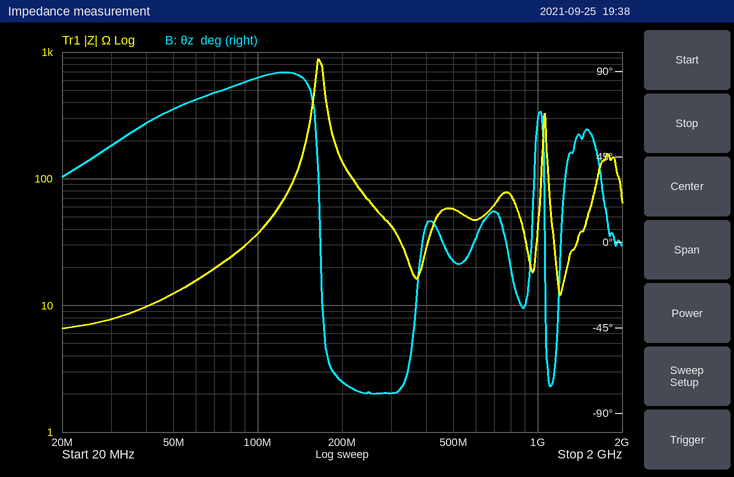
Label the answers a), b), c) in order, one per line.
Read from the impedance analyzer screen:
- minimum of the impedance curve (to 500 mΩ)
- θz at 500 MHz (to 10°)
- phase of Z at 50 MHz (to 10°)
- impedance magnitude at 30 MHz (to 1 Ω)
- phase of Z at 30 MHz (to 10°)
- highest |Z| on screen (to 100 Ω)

a) 6.5 Ω
b) -10°
c) 70°
d) 8 Ω
e) 50°
f) 900 Ω
